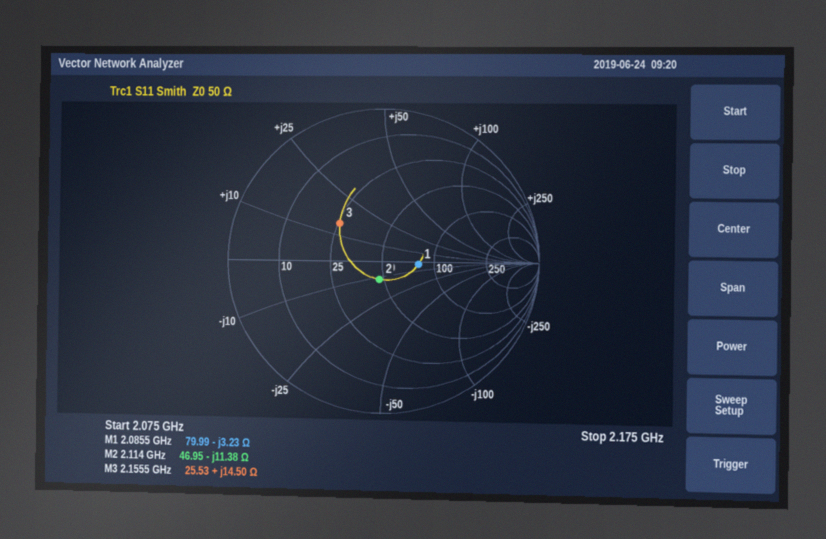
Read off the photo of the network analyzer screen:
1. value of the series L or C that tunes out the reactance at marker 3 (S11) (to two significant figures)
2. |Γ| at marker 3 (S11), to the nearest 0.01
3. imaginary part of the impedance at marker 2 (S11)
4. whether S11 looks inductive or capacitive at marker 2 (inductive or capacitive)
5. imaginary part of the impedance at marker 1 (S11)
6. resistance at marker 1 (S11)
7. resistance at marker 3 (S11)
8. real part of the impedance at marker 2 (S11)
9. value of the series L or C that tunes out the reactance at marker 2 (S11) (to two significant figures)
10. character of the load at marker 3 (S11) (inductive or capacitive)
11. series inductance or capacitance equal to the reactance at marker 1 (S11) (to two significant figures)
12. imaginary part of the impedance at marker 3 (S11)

5.1 pF
0.37
-11.38 Ω
capacitive
-3.23 Ω
79.99 Ω
25.53 Ω
46.95 Ω
860 pH
inductive
24 pF
+14.50 Ω
